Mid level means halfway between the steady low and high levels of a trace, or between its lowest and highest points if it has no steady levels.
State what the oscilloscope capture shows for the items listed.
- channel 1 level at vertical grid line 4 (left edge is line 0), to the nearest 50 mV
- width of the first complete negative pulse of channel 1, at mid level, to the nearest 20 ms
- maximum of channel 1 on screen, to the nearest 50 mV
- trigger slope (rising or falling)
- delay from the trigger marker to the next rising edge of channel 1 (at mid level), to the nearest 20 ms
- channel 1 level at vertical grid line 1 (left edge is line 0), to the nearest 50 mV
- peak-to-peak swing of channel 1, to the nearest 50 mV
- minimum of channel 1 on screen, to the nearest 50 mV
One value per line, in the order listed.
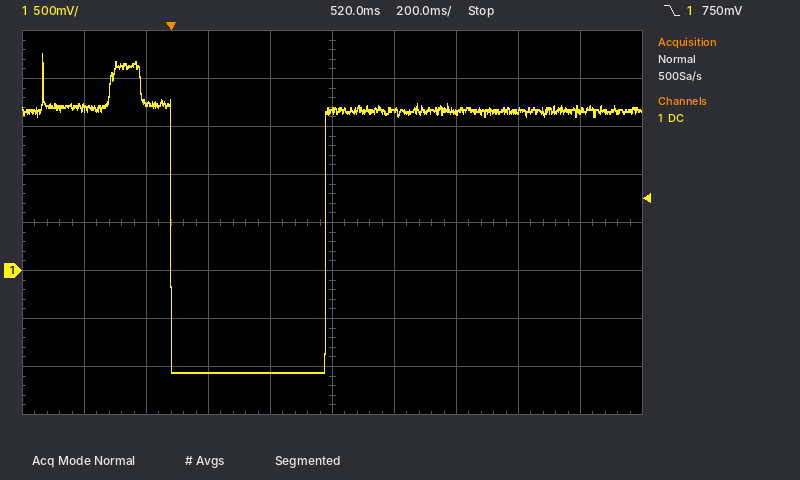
-1.05 V
500 ms
2.25 V
falling
500 ms
1.70 V
3.30 V
-1.05 V
